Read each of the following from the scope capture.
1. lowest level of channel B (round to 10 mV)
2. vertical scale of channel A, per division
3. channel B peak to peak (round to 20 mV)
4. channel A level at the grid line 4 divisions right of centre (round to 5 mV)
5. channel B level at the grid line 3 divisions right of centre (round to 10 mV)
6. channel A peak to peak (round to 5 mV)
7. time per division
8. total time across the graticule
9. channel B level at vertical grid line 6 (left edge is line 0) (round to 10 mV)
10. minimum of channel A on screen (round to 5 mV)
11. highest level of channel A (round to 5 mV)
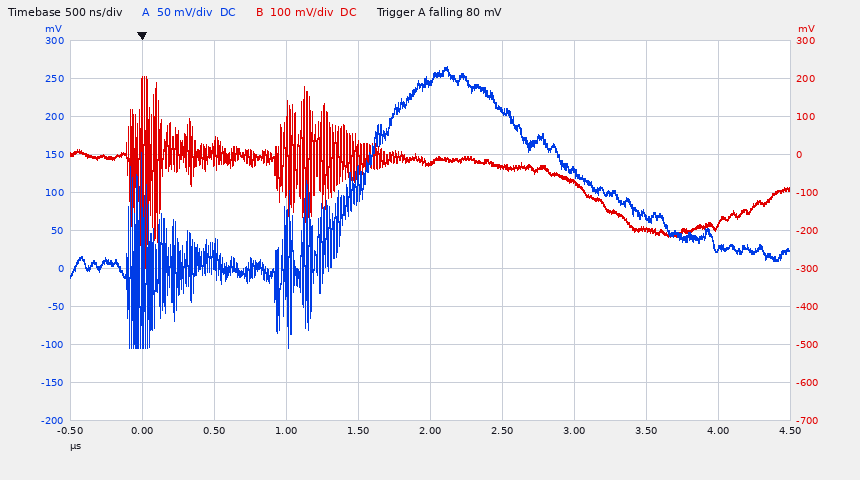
-300 mV
50 mV
500 mV
25 mV
-200 mV
370 mV
500 ns
5 µs
-30 mV
-105 mV
265 mV
